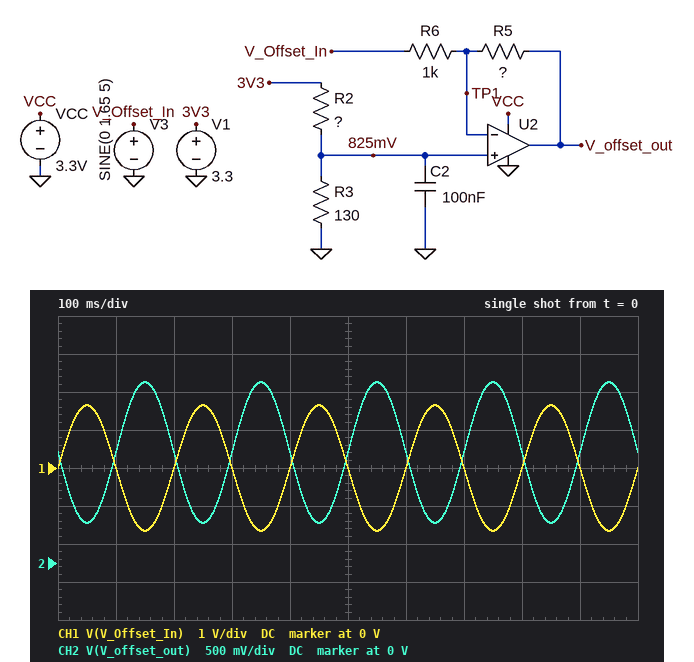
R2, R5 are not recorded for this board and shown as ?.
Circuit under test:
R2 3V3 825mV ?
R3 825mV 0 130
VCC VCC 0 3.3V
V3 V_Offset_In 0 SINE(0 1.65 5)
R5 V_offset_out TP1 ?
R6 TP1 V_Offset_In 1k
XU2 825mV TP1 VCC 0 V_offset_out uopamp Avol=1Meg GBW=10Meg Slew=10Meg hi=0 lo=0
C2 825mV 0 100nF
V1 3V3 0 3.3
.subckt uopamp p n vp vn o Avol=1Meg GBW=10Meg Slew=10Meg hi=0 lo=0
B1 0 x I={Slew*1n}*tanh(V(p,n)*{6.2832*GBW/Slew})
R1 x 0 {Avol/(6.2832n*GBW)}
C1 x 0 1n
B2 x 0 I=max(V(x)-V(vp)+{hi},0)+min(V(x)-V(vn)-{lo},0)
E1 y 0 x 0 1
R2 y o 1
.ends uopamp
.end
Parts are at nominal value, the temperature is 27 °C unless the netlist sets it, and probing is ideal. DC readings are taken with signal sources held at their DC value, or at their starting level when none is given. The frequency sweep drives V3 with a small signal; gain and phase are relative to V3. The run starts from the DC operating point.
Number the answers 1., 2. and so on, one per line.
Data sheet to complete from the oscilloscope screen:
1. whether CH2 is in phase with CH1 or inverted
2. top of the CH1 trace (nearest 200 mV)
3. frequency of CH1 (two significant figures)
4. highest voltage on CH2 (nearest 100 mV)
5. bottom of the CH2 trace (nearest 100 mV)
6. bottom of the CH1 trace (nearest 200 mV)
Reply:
1. inverted
2. 1.6 V
3. 5.0 Hz
4. 2.4 V
5. 500 mV
6. -1.6 V
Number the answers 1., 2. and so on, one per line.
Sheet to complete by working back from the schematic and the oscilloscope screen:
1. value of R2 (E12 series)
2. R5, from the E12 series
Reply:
1. 330 Ω
2. 560 Ω
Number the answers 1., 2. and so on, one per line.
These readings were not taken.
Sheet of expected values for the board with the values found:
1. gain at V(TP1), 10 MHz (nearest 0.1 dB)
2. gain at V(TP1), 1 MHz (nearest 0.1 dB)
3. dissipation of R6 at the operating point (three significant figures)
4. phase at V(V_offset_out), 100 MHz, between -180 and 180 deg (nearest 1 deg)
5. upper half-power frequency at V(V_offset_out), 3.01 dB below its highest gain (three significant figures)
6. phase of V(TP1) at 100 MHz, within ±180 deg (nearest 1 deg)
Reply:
1. -10.4 dB
2. -25.1 dB
3. 870 µW
4. 93 deg
5. 6.41 MHz
6. 4 deg
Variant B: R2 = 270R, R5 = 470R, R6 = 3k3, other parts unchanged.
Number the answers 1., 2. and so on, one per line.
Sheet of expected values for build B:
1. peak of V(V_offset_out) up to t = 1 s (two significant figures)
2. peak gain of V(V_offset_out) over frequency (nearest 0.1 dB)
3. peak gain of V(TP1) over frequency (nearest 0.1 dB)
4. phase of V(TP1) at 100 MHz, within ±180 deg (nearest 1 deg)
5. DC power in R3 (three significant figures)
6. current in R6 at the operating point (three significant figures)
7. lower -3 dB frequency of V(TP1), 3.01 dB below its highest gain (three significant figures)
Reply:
1. 1.5 V
2. -16.9 dB
3. -18.1 dB
4. 5 deg
5. 8.85 mW
6. 325 µA
7. 8.75 MHz
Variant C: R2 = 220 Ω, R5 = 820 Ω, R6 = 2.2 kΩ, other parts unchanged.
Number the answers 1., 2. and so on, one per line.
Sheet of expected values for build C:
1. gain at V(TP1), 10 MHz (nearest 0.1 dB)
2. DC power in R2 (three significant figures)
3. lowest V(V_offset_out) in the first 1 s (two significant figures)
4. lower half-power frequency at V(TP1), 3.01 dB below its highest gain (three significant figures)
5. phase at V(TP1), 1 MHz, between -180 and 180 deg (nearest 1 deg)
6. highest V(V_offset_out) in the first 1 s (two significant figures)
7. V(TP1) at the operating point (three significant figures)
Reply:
1. -13.2 dB
2. 19.6 mW
3. 1.1 V
4. 7.28 MHz
5. 82 deg
6. 2.3 V
7. 1.23 V
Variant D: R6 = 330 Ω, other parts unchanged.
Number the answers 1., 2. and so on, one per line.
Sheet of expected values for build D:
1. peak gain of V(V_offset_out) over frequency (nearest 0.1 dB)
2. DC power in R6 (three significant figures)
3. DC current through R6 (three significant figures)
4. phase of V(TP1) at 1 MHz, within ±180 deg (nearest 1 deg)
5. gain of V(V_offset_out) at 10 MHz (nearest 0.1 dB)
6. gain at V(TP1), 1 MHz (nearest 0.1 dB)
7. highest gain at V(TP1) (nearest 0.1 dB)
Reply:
1. 4.6 dB
2. 2.64 mW
3. 2.83 mA
4. 75 deg
5. -4.6 dB
6. -15.7 dB
7. -4.0 dB
